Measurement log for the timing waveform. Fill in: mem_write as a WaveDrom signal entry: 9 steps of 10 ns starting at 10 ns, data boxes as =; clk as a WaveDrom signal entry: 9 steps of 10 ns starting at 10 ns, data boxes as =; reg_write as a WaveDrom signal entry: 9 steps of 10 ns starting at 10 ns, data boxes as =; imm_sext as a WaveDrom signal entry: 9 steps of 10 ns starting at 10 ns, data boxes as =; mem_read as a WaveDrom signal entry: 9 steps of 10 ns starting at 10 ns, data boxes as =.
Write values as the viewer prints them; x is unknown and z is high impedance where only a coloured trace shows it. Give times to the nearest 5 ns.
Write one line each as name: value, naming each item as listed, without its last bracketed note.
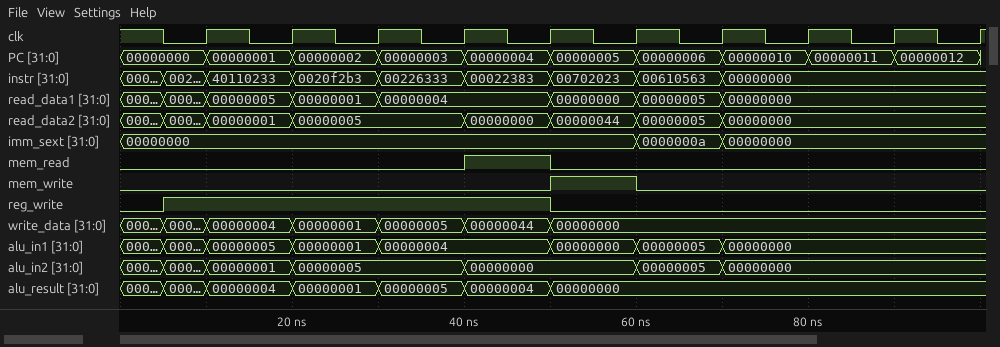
mem_write as a WaveDrom signal entry: 9 steps of 10 ns starting at 10 ns, data boxes as =: {name: 'mem_write', wave: '0...10...'}
clk as a WaveDrom signal entry: 9 steps of 10 ns starting at 10 ns, data boxes as =: {name: 'clk', wave: 'p........'}
reg_write as a WaveDrom signal entry: 9 steps of 10 ns starting at 10 ns, data boxes as =: {name: 'reg_write', wave: '1...0....'}
imm_sext as a WaveDrom signal entry: 9 steps of 10 ns starting at 10 ns, data boxes as =: {name: 'imm_sext', wave: '=....==..', data: '00000000 0000000a 00000000'}
mem_read as a WaveDrom signal entry: 9 steps of 10 ns starting at 10 ns, data boxes as =: {name: 'mem_read', wave: '0..10....'}
